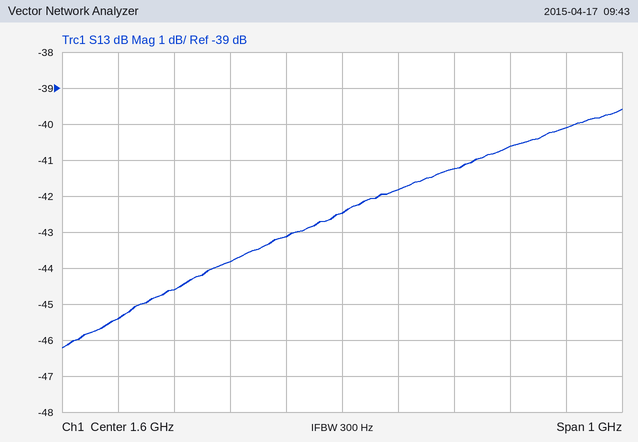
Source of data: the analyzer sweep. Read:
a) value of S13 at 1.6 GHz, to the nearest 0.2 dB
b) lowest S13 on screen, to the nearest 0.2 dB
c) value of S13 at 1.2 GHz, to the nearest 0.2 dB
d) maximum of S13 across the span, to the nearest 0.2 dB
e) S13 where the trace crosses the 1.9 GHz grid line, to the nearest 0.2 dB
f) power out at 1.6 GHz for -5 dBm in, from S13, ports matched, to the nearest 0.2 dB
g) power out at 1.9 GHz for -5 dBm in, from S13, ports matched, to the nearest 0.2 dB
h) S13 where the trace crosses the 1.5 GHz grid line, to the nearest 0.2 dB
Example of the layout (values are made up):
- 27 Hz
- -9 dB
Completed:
- -42.4 dB
- -46.2 dB
- -45.4 dB
- -39.6 dB
- -40.6 dB
- -47.4 dBm
- -45.6 dBm
- -43.2 dB
